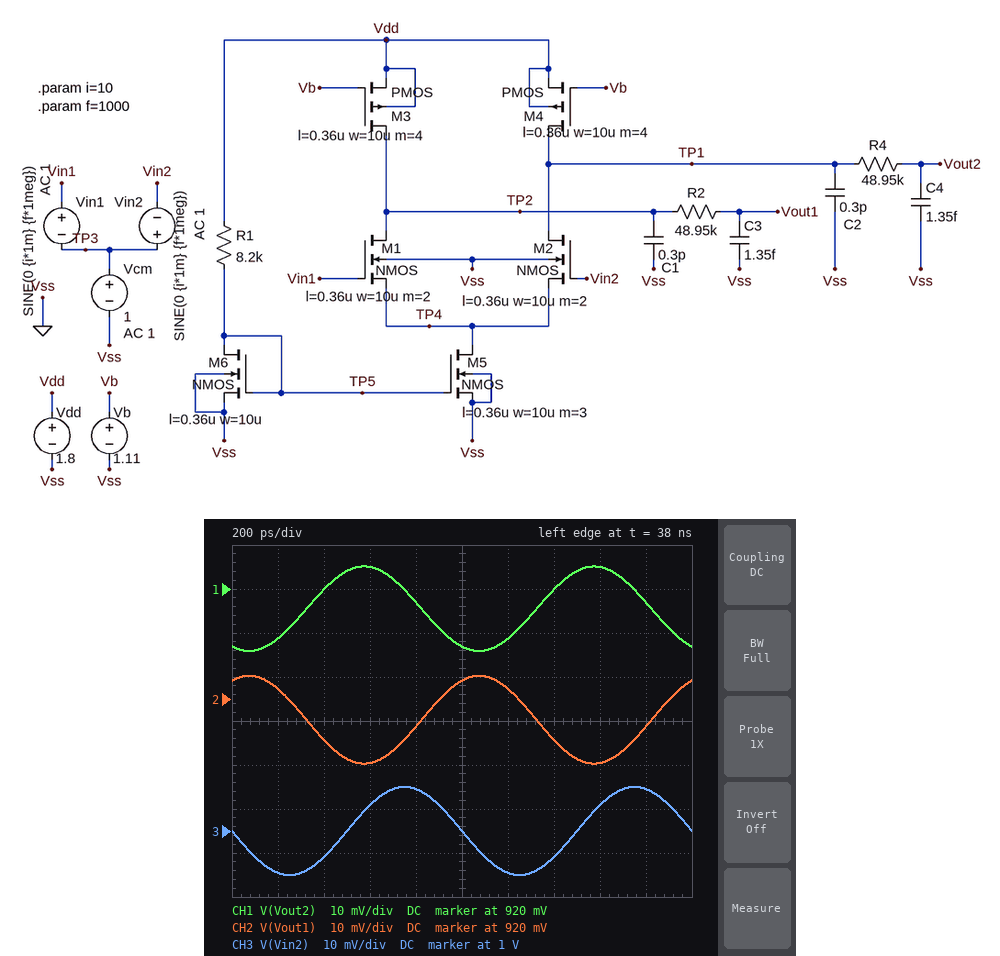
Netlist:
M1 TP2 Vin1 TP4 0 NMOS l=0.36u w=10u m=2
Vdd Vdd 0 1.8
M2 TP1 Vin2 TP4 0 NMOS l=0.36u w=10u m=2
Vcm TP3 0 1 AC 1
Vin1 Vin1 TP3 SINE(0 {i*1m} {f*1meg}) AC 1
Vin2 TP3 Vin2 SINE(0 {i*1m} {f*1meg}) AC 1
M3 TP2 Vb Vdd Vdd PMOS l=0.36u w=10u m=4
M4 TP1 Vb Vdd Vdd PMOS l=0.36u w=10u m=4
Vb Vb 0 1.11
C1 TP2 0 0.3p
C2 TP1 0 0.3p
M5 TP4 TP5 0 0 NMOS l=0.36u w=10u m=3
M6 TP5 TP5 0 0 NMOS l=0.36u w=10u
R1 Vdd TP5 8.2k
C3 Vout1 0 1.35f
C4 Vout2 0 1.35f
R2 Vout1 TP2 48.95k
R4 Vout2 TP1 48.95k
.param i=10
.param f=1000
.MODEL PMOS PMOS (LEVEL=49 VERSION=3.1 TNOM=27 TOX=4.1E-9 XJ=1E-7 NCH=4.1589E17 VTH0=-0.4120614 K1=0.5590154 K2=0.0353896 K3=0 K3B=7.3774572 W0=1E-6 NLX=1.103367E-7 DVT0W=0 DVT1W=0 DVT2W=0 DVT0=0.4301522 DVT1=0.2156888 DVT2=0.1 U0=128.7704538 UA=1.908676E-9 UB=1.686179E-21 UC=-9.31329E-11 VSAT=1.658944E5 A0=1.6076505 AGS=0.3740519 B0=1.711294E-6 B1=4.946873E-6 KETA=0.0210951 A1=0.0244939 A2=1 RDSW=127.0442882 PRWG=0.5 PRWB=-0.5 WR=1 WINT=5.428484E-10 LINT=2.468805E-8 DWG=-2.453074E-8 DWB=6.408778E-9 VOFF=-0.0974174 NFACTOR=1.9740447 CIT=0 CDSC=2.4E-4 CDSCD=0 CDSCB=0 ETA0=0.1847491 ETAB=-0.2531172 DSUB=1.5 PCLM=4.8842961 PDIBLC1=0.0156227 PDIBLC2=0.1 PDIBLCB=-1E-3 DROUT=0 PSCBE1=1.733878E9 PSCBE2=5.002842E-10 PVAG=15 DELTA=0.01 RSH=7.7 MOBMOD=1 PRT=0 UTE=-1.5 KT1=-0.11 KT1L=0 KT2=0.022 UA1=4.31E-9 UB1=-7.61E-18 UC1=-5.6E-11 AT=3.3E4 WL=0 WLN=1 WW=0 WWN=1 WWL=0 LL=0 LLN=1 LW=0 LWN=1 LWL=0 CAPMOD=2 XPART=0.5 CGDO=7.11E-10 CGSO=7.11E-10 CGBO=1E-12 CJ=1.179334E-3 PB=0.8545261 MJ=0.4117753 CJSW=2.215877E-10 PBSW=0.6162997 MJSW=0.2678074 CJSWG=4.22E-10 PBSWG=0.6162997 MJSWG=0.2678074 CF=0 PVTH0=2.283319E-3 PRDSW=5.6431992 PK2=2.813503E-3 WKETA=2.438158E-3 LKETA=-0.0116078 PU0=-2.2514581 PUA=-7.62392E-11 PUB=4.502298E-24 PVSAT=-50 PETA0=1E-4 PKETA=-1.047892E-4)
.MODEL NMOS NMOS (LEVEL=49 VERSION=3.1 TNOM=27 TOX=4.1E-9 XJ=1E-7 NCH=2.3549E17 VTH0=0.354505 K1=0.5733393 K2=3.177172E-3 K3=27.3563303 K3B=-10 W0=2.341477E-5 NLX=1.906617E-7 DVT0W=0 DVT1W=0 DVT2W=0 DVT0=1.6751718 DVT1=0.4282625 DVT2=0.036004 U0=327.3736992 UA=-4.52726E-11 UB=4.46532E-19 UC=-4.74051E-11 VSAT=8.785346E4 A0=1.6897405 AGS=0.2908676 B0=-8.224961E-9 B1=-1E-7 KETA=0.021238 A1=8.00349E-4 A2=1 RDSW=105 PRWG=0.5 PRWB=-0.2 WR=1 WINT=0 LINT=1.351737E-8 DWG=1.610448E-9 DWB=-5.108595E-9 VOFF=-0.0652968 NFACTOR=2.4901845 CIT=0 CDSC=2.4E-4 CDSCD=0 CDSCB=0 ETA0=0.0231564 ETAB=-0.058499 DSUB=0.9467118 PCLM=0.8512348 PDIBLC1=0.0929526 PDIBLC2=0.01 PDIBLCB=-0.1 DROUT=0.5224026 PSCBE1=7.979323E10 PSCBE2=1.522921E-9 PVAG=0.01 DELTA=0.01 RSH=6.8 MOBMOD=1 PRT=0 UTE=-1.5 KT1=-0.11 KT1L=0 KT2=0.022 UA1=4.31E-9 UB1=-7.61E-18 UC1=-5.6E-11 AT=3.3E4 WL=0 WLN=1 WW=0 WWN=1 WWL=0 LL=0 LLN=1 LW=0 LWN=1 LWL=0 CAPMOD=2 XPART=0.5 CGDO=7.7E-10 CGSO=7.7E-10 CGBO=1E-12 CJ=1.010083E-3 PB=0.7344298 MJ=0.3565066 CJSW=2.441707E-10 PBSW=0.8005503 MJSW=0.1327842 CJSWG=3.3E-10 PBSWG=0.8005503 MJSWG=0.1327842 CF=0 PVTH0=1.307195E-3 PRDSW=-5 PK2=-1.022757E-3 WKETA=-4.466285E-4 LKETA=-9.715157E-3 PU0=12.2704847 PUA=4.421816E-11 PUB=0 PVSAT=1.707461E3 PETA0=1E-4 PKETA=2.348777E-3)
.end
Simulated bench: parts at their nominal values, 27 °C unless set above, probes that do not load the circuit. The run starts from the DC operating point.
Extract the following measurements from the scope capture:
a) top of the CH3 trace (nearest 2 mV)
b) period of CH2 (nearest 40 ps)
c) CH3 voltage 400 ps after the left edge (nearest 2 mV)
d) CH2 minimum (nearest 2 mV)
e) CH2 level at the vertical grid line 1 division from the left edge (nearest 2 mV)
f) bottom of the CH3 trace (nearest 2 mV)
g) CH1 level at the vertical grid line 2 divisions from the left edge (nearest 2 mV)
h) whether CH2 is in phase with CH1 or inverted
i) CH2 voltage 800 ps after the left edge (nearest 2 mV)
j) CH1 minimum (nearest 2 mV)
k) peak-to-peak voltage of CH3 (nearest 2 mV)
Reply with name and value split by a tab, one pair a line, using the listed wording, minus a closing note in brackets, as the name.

top of the CH3 trace	1.010 V
period of CH2	1.00 ns
CH3 voltage 400 ps after the left edge	994 mV
CH2 minimum	906 mV
CH2 level at the vertical grid line 1 division from the left edge	922 mV
bottom of the CH3 trace	990 mV
CH1 level at the vertical grid line 2 divisions from the left edge	920 mV
whether CH2 is in phase with CH1 or inverted	inverted
CH2 voltage 800 ps after the left edge	914 mV
CH1 minimum	906 mV
peak-to-peak voltage of CH3	20 mV
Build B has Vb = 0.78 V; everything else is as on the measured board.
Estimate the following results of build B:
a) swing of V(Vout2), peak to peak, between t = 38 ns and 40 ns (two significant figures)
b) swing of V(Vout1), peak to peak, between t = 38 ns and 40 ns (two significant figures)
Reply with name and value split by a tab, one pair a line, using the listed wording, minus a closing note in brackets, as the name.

swing of V(Vout2), peak to peak, between t = 38 ns and 40 ns	9.6 mV
swing of V(Vout1), peak to peak, between t = 38 ns and 40 ns	9.7 mV
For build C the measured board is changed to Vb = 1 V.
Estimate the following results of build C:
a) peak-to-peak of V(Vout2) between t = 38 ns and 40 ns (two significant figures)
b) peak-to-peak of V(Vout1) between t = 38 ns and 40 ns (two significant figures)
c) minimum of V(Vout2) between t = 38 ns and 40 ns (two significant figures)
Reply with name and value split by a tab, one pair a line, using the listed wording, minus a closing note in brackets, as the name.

peak-to-peak of V(Vout2) between t = 38 ns and 40 ns	14 mV
peak-to-peak of V(Vout1) between t = 38 ns and 40 ns	15 mV
minimum of V(Vout2) between t = 38 ns and 40 ns	1.7 V
